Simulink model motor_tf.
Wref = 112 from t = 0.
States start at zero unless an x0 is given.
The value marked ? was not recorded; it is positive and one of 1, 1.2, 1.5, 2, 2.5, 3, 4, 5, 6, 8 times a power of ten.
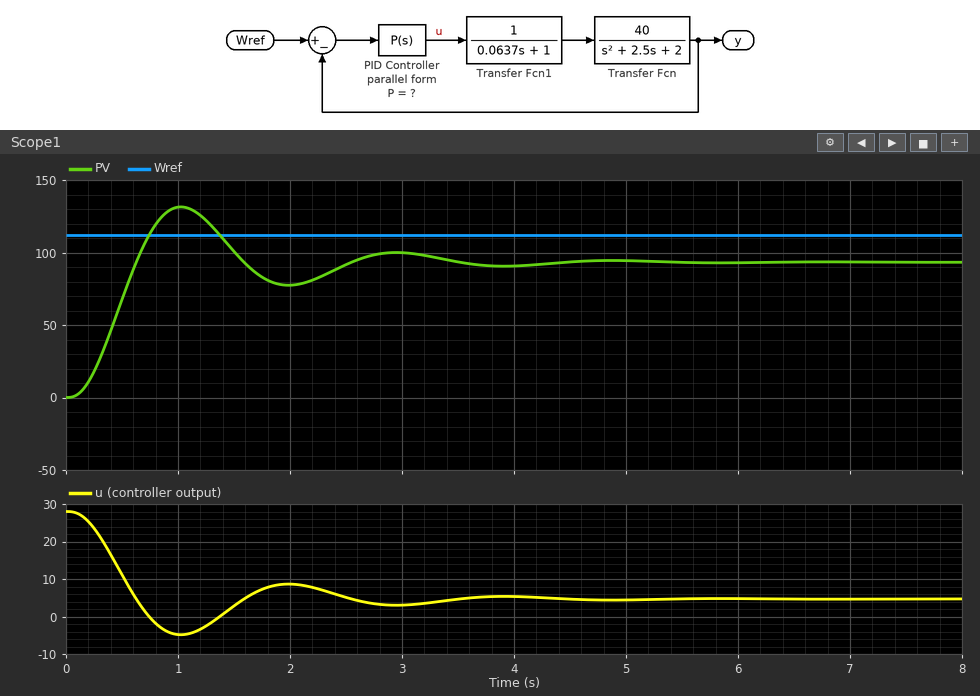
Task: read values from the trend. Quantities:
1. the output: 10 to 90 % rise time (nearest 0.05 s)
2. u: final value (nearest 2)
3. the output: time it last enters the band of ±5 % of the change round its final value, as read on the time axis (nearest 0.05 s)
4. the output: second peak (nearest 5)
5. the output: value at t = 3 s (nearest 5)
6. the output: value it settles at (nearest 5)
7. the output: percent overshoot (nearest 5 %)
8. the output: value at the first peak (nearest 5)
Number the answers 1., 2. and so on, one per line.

1. 0.40 s
2. 4
3. 3.20 s
4. 100
5. 100
6. 95
7. 40 %
8. 130
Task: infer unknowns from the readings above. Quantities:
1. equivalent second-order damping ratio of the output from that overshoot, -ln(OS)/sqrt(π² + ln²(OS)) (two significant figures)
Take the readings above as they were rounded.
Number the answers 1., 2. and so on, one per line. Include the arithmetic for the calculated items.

1. ln(0.4) = -0.916; 0.916 / sqrt(9.870 + 0.840) = 0.28
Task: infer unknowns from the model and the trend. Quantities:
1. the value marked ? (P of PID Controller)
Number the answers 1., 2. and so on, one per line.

1. 0.25
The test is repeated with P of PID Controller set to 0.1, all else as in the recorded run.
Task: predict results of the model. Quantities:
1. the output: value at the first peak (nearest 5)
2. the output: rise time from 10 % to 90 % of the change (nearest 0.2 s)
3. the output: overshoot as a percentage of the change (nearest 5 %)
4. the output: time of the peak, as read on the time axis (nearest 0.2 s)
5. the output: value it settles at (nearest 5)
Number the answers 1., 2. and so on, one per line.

1. 90
2. 0.6 s
3. 20 %
4. 1.6 s
5. 75
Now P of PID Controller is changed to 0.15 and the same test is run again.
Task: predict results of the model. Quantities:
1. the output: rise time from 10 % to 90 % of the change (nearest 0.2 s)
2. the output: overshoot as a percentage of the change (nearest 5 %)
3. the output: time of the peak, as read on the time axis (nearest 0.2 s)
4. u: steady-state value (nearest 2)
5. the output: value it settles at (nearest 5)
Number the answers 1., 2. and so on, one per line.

1. 0.6 s
2. 30 %
3. 1.2 s
4. 4
5. 85
